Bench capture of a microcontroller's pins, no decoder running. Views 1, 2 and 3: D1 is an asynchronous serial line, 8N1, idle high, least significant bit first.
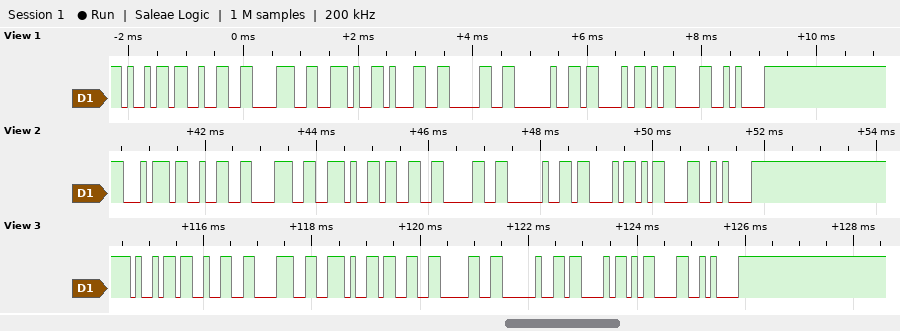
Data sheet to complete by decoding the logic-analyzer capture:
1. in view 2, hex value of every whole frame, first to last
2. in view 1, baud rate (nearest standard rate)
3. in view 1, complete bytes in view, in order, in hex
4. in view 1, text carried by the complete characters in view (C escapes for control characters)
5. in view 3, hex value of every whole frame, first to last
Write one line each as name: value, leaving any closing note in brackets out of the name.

in view 2, hex value of every whole frame, first to last: 74 32 38 2E 33 30 20 43 0D 0A
in view 1, baud rate: 9600 baud
in view 1, complete bytes in view, in order, in hex: 0x69 0x32 0x38 0x2E 0x31 0x30 0x20 0x43 0x0D 0x0A
in view 1, text carried by the complete characters in view: "i28.10 C\r\n"
in view 3, hex value of every whole frame, first to last: 69 32 38 2E 33 30 20 43 0D 0A
